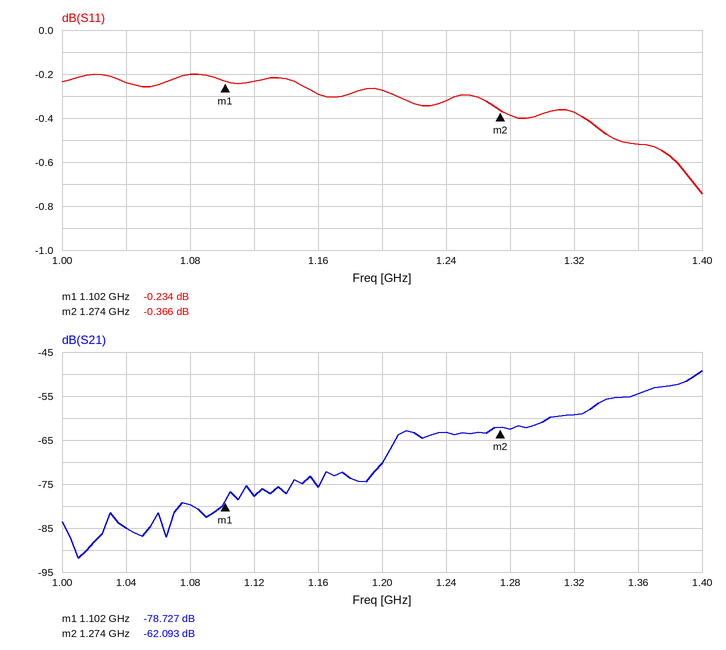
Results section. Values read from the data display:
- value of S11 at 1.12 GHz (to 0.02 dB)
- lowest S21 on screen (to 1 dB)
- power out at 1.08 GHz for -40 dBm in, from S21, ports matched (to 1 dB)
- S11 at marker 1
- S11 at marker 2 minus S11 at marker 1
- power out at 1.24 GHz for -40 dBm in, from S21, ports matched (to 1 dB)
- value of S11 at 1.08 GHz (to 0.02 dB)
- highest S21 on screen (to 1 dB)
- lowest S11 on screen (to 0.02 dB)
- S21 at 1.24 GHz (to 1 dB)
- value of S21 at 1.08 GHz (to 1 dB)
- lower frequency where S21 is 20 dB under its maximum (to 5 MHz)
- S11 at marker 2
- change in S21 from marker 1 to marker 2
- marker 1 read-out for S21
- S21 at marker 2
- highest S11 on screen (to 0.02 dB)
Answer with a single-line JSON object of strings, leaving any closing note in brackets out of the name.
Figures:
{"value of S11 at 1.12 GHz": "-0.24 dB", "lowest S21 on screen": "-92 dB", "power out at 1.08 GHz for -40 dBm in, from S21, ports matched": "-120 dBm", "S11 at marker 1": "-0.234 dB", "S11 at marker 2 minus S11 at marker 1": "-0.132 dB", "power out at 1.24 GHz for -40 dBm in, from S21, ports matched": "-103 dBm", "value of S11 at 1.08 GHz": "-0.20 dB", "highest S21 on screen": "-49 dB", "lowest S11 on screen": "-0.74 dB", "S21 at 1.24 GHz": "-63 dB", "value of S21 at 1.08 GHz": "-80 dB", "lower frequency where S21 is 20 dB under its maximum": "1.200 GHz", "S11 at marker 2": "-0.366 dB", "change in S21 from marker 1 to marker 2": "16.634 dB", "marker 1 read-out for S21": "-78.727 dB", "S21 at marker 2": "-62.093 dB", "highest S11 on screen": "-0.20 dB"}
